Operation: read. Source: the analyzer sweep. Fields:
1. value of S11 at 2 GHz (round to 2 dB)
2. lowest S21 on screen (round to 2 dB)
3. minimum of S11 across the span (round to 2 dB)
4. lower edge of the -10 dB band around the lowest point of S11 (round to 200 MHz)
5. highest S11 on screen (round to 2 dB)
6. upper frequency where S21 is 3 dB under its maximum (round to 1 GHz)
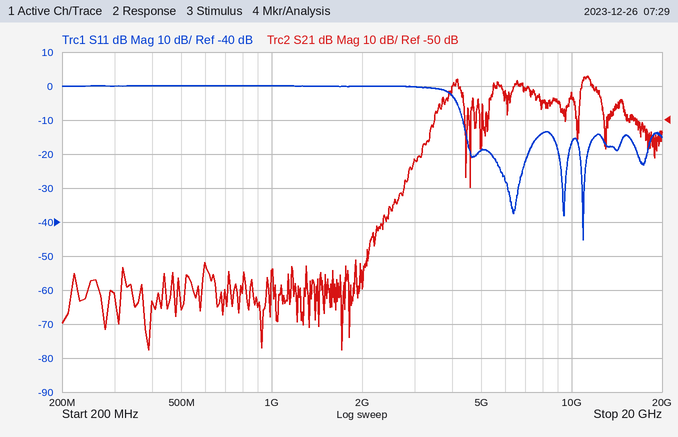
0 dB
-118 dB
-46 dB
4.4 GHz
0 dB
12 GHz
